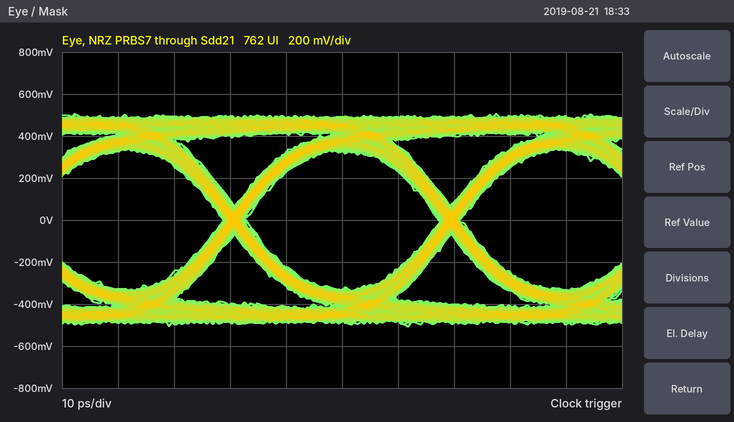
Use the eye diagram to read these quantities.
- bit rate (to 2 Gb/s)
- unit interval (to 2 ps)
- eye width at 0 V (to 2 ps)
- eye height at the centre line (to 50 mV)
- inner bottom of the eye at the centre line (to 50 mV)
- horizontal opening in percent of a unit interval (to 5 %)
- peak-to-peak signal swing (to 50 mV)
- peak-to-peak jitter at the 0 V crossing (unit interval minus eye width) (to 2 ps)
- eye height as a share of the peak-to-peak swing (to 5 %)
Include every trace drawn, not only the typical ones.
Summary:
26 Gb/s
38 ps
34 ps
650 mV
-350 mV
90 %
1.00 V
4 ps
65 %
